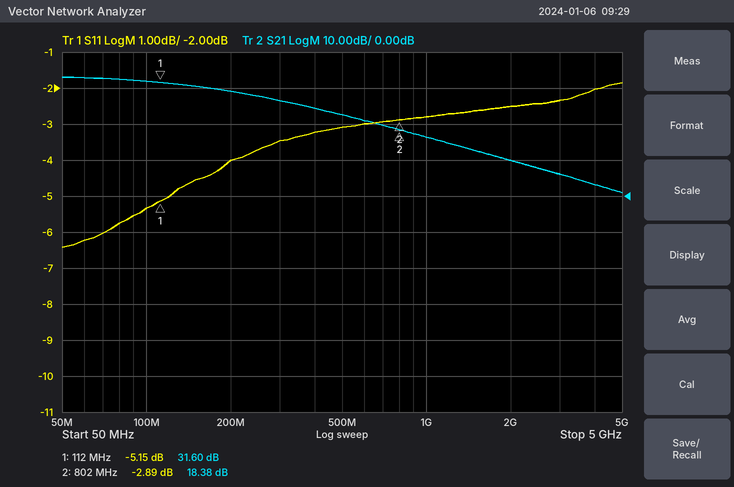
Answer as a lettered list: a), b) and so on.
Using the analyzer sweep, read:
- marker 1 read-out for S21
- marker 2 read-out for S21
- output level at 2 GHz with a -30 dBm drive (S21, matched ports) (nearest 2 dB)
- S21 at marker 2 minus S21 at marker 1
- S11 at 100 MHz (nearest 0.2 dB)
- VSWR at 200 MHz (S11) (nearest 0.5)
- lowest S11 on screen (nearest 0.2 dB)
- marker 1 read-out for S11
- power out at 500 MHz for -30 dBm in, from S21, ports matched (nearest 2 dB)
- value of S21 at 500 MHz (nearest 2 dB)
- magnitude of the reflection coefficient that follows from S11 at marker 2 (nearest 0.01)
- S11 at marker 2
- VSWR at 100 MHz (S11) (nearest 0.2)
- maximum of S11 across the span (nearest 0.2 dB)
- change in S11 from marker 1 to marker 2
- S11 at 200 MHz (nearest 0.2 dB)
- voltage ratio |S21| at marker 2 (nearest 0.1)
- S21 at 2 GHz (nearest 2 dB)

a) 31.60 dB
b) 18.38 dB
c) -20 dBm
d) -13.22 dB
e) -5.4 dB
f) 4.5
g) -6.4 dB
h) -5.15 dB
i) -8 dBm
j) 22 dB
k) 0.72
l) -2.89 dB
m) 3.4
n) -1.8 dB
o) 2.26 dB
p) -4.0 dB
q) 8.3
r) 10 dB
